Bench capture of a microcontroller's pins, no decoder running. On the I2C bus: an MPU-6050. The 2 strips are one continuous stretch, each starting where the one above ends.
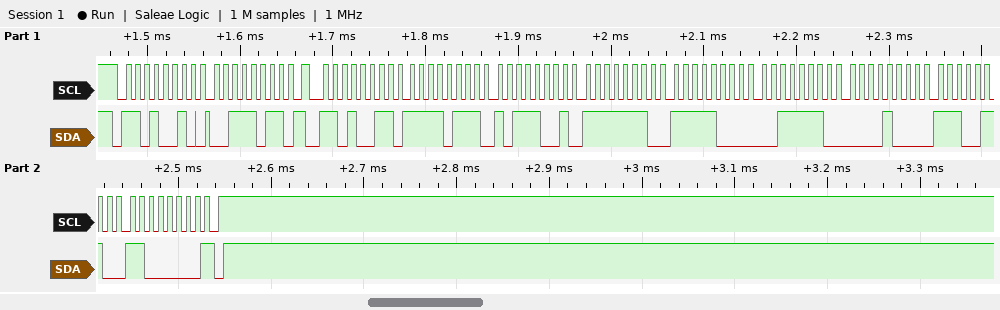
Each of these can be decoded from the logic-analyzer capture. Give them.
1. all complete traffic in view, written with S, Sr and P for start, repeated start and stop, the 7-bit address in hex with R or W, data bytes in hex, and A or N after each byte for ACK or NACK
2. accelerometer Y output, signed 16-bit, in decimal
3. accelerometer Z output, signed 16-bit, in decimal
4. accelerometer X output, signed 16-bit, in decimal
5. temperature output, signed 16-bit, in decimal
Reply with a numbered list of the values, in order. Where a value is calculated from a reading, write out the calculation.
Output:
1. S 69W A 3B A Sr 69R A F7 A B9 A FE A F8 A 3E A 08 A E6 A C0 N P
2. 0xFEF8 = -264
3. 0x3E08 = 15880
4. 0xF7B9 = -2119
5. 0xE6C0 = -6464
